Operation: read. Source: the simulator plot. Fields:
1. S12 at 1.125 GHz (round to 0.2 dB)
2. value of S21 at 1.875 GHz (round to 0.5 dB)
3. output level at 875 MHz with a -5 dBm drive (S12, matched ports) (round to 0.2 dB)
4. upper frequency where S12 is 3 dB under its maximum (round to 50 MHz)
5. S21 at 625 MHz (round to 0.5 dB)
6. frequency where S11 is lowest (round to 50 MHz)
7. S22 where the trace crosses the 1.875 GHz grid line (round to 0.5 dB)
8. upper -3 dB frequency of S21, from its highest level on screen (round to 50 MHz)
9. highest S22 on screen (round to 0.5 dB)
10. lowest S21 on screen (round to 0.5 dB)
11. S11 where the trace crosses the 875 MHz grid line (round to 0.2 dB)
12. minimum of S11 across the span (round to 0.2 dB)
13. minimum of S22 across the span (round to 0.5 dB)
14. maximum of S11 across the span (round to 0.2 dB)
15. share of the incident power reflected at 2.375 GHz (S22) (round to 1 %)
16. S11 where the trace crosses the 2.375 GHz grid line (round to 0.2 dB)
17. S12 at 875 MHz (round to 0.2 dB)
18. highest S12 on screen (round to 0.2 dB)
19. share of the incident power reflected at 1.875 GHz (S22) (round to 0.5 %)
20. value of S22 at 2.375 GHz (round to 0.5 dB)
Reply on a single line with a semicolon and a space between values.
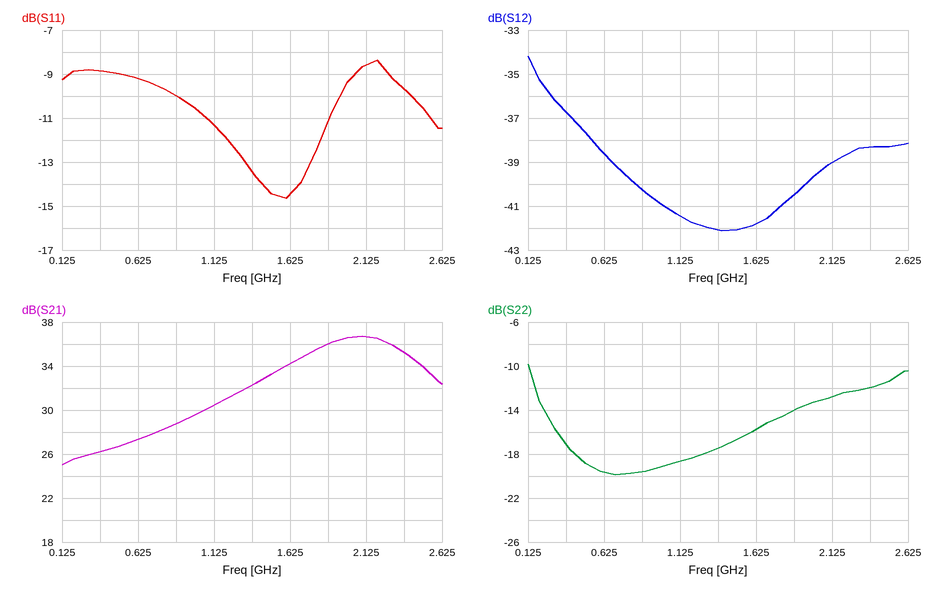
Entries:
-41.4 dB; 36.0 dB; -45.2 dBm; 450 MHz; 27.5 dB; 1.60 GHz; -14.0 dB; 2.50 GHz; -10.0 dB; 25.0 dB; -10.0 dB; -14.6 dB; -20.0 dB; -8.4 dB; 6 %; -9.6 dB; -40.2 dB; -34.2 dB; 4.0 %; -12.0 dB
